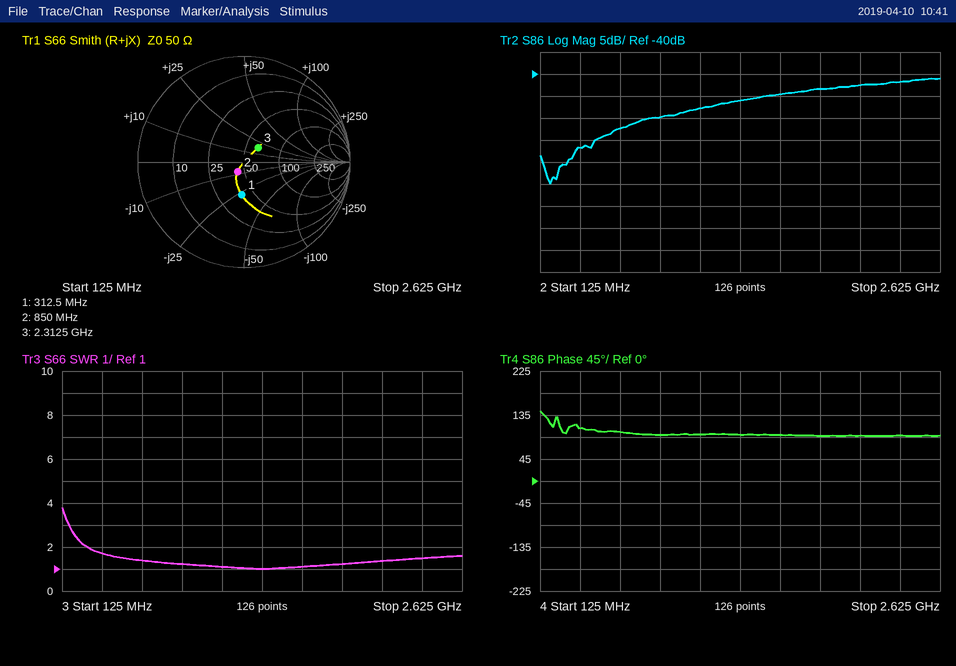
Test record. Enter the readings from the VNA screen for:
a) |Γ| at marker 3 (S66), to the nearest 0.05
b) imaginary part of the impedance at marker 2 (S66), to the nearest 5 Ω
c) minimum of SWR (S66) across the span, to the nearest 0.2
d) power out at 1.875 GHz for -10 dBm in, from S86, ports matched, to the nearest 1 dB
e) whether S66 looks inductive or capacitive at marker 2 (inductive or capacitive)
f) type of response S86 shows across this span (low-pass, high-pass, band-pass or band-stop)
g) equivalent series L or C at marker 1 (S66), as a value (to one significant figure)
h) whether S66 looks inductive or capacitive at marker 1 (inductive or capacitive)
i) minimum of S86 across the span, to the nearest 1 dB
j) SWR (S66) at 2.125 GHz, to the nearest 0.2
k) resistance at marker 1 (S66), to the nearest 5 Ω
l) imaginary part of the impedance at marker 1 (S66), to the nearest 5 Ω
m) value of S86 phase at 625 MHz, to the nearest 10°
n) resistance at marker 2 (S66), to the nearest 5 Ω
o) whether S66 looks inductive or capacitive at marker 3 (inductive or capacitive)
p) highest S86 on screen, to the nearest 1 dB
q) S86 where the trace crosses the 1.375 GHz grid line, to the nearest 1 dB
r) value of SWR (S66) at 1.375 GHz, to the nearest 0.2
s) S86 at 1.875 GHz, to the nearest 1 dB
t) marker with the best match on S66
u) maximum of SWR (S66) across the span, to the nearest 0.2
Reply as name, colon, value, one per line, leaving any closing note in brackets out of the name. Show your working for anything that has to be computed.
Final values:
|Γ| at marker 3 (S66), to the nearest 0.05: 0.20
imaginary part of the impedance at marker 2 (S66), to the nearest 5 Ω: -10 Ω
minimum of SWR (S66) across the span, to the nearest 0.2: 1.0
power out at 1.875 GHz for -10 dBm in, from S86, ports matched, to the nearest 1 dB: -10 dBm + (-43 dB) = -53 dBm
whether S66 looks inductive or capacitive at marker 2: capacitive
type of response S86 shows across this span: high-pass
equivalent series L or C at marker 1 (S66), as a value: C = 1/(2π × 312.5 MHz × 25 Ω) ≈ 20 pF
whether S66 looks inductive or capacitive at marker 1: capacitive
minimum of S86 across the span, to the nearest 1 dB: -65 dB
SWR (S66) at 2.125 GHz, to the nearest 0.2: 1.4
resistance at marker 1 (S66), to the nearest 5 Ω: 40 Ω
imaginary part of the impedance at marker 1 (S66), to the nearest 5 Ω: -25 Ω
value of S86 phase at 625 MHz, to the nearest 10°: 100°
resistance at marker 2 (S66), to the nearest 5 Ω: 45 Ω
whether S66 looks inductive or capacitive at marker 3: inductive
highest S86 on screen, to the nearest 1 dB: -41 dB
S86 where the trace crosses the 1.375 GHz grid line, to the nearest 1 dB: -46 dB
value of SWR (S66) at 1.375 GHz, to the nearest 0.2: 1.0
S86 at 1.875 GHz, to the nearest 1 dB: -43 dB
marker with the best match on S66: marker 2
maximum of SWR (S66) across the span, to the nearest 0.2: 3.8
